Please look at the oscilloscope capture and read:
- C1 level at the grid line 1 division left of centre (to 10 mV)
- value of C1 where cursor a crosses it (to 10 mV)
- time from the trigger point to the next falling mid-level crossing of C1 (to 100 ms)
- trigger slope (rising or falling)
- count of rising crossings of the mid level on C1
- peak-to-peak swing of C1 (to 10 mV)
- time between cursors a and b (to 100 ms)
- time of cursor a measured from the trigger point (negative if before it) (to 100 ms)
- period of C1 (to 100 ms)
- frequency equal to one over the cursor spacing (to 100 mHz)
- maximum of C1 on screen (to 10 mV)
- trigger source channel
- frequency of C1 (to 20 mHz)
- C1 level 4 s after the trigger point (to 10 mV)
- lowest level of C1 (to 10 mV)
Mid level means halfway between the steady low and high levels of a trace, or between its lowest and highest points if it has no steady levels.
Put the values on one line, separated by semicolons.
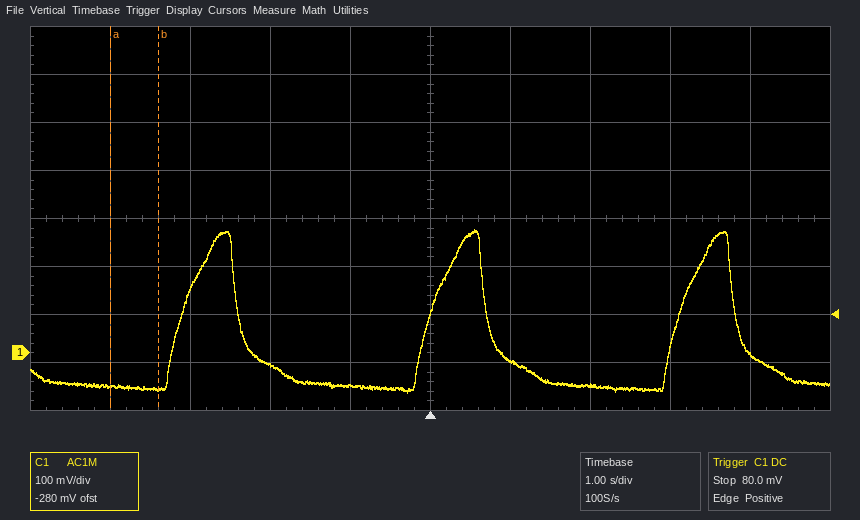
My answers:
-70 mV; -70 mV; 700 ms; rising; 3; 340 mV; 600 ms; -4.0 s; 3.1 s; 1.7 Hz; 260 mV; C1; 320 mHz; 0 mV; -80 mV
